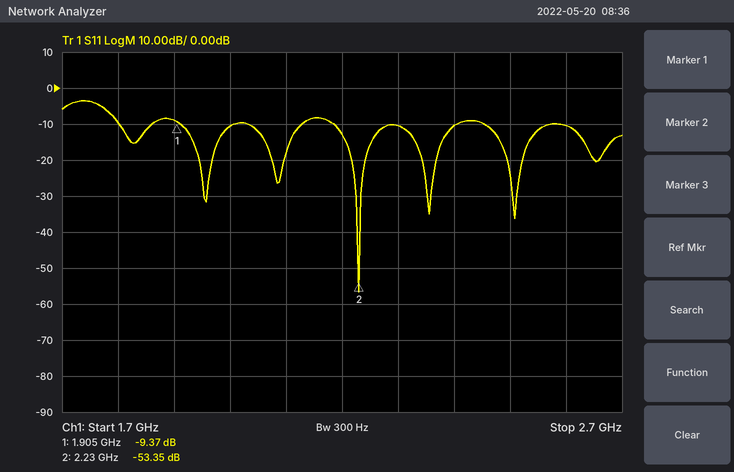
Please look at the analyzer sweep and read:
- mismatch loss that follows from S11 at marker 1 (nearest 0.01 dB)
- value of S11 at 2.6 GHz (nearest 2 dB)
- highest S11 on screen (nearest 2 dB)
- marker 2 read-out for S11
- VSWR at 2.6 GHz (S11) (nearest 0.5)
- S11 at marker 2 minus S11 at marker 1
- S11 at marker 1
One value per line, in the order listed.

0.53 dB
-10 dB
-4 dB
-53.35 dB
2.0
-43.98 dB
-9.37 dB
